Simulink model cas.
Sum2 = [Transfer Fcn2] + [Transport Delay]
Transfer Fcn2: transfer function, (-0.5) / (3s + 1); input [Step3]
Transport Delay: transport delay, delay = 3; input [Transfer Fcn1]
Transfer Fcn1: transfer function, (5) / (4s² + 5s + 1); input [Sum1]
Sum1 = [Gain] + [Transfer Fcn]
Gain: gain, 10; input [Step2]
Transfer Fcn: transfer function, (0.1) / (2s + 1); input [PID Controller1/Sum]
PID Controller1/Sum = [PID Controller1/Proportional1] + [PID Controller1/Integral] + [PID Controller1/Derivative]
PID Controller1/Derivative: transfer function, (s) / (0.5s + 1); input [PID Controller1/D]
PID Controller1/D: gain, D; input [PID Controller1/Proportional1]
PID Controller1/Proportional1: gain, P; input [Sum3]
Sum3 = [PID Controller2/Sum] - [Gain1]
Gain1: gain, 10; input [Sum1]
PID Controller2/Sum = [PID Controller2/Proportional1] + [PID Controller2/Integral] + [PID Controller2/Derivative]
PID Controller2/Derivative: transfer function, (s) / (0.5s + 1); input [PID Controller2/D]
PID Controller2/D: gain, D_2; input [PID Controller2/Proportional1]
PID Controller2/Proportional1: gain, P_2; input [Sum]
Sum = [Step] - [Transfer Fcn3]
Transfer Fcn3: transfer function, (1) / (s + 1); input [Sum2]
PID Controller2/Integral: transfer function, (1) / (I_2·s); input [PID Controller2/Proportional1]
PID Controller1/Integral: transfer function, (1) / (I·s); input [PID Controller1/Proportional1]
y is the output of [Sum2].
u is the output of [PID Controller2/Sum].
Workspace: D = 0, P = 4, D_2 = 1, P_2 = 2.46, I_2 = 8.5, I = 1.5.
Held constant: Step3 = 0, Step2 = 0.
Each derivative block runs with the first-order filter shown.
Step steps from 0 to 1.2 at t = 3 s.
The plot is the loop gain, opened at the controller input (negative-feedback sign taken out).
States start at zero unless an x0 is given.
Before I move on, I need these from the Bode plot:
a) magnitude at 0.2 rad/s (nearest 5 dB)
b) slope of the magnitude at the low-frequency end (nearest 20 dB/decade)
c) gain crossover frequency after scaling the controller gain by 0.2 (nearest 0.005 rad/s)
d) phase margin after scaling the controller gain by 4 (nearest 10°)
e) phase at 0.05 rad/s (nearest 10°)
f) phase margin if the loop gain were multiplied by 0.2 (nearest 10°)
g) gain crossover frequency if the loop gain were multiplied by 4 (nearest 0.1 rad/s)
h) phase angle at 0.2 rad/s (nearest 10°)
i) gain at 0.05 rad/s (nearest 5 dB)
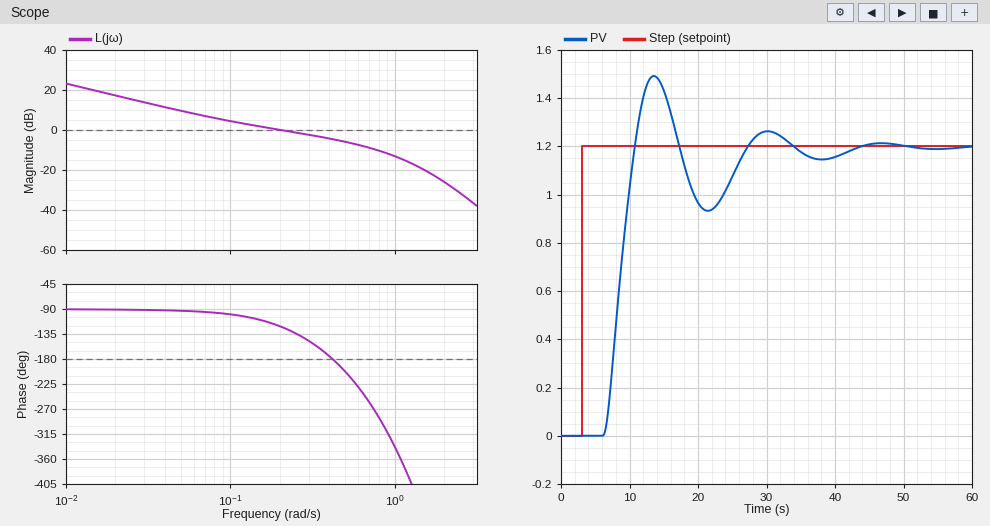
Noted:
0 dB
-20 dB/decade
0.030 rad/s
-140°
-90°
90°
0.9 rad/s
-120°
10 dB
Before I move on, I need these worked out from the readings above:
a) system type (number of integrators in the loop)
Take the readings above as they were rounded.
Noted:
1
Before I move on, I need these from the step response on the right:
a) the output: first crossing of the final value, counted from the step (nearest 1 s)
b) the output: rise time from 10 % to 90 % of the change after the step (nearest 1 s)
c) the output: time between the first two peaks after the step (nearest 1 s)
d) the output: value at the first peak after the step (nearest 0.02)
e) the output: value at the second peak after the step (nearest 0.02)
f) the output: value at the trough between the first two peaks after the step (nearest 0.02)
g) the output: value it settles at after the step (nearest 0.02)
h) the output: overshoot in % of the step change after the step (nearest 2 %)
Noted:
8 s
3 s
17 s
1.50
1.26
0.94
1.20
24 %
